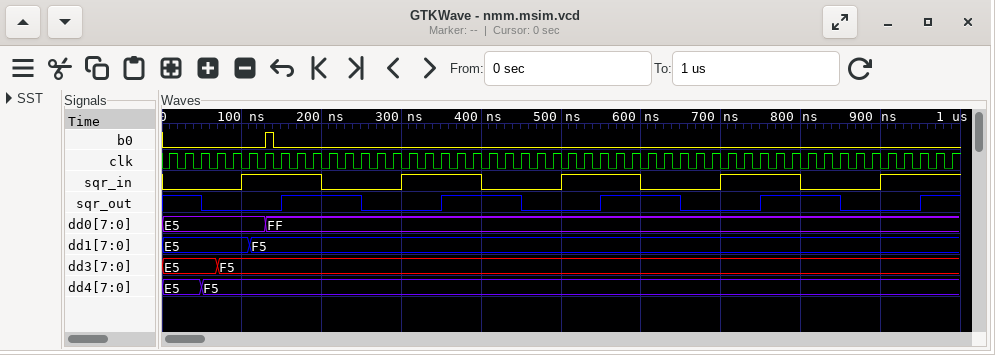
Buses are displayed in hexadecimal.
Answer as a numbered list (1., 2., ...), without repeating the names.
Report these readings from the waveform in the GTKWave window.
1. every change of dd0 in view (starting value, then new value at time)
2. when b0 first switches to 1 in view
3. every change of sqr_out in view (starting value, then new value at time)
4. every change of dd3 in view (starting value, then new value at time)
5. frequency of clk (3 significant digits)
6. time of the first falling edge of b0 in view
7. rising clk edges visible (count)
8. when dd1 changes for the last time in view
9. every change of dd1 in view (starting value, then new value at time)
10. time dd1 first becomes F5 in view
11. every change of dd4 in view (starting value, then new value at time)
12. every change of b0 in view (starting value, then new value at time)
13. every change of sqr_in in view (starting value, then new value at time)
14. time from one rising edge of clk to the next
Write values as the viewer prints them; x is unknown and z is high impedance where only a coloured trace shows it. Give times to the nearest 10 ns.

1. E5, FF at 130 ns
2. 130 ns
3. 1, 0 at 50 ns, 1 at 150 ns, 0 at 250 ns, 1 at 350 ns, 0 at 450 ns, 1 at 550 ns, 0 at 650 ns, 1 at 750 ns, 0 at 850 ns, 1 at 950 ns
4. E5, F5 at 70 ns
5. 50.0 MHz
6. 140 ns
7. 50
8. 110 ns
9. E5, F5 at 110 ns
10. 110 ns
11. E5, F5 at 50 ns
12. 0, 1 at 130 ns, 0 at 140 ns
13. 0, 1 at 100 ns, 0 at 200 ns, 1 at 300 ns, 0 at 400 ns, 1 at 500 ns, 0 at 600 ns, 1 at 700 ns, 0 at 800 ns, 1 at 900 ns
14. 20 ns
